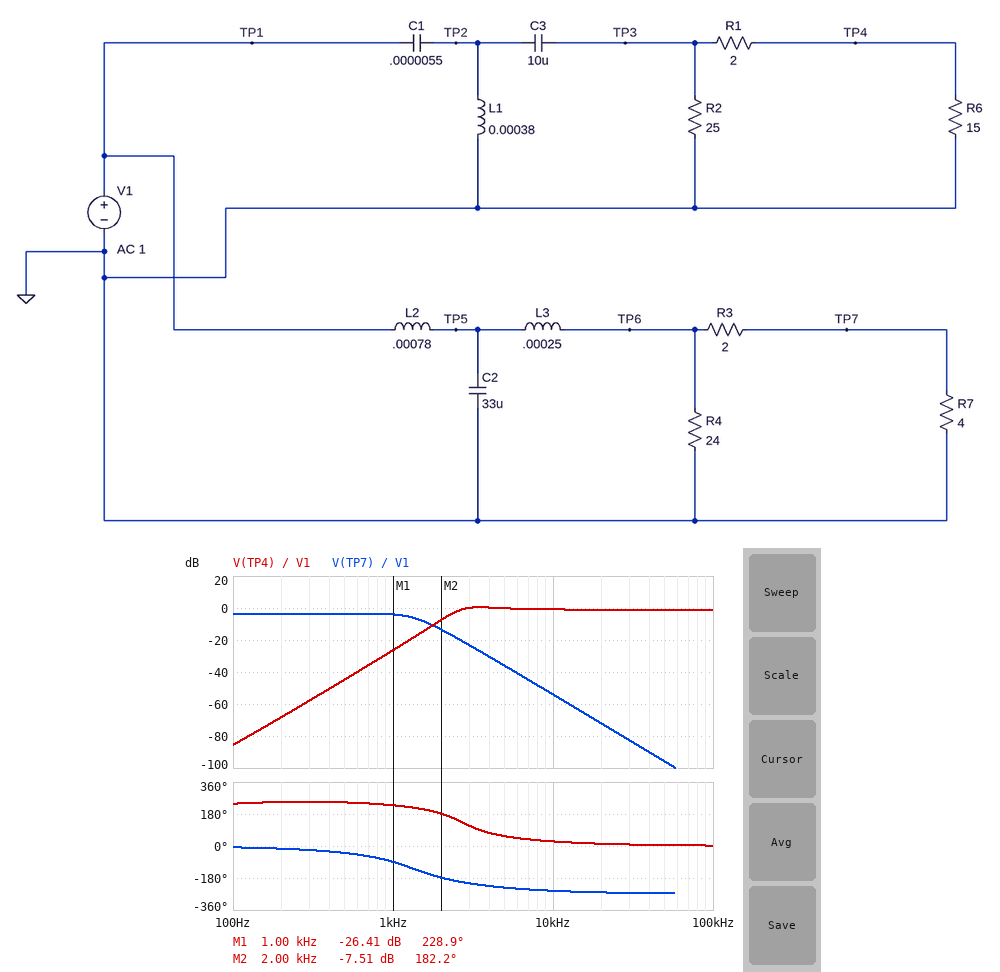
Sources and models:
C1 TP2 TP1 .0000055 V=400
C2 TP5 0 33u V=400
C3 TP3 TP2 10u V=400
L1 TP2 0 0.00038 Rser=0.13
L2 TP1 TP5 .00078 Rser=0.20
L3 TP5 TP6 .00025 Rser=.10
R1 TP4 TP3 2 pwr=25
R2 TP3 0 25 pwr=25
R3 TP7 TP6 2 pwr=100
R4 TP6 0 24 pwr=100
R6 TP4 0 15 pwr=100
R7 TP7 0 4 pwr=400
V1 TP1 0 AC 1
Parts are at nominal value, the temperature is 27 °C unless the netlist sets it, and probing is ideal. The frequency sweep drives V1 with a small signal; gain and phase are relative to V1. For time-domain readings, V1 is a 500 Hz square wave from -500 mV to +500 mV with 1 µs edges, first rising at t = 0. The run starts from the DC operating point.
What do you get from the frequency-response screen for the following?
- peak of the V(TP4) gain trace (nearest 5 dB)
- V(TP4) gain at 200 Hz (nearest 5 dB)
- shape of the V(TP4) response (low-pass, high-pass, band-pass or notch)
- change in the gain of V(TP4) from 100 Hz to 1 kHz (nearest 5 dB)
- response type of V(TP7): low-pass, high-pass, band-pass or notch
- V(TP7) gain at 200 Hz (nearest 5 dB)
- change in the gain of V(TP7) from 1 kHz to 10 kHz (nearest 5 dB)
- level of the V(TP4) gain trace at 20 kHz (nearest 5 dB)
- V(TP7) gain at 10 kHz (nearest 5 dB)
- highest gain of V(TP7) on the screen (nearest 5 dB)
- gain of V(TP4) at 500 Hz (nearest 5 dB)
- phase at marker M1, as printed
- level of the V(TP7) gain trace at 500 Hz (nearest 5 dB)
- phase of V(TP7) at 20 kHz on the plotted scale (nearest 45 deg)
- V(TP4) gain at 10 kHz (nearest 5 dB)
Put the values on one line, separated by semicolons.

0 dB; -70 dB; high-pass; 60 dB; low-pass; -5 dB; -50 dB; 0 dB; -55 dB; -5 dB; -45 dB; 228.9 deg; -5 dB; -270 deg; 0 dB
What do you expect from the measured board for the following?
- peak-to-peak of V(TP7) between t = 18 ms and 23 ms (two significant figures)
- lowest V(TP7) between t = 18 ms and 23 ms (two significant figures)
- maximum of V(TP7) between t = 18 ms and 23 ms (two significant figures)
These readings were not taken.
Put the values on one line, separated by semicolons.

770 mV; -380 mV; 380 mV
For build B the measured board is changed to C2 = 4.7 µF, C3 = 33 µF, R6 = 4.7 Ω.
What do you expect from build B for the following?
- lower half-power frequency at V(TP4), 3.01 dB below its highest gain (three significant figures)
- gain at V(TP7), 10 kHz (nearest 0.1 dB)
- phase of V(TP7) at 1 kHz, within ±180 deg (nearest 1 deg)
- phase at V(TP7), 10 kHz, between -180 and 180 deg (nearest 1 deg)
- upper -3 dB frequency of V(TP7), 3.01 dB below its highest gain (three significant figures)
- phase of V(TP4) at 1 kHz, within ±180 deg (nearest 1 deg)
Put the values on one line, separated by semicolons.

4.21 kHz; -34.8 dB; -55 deg; 112 deg; 887 Hz; -161 deg
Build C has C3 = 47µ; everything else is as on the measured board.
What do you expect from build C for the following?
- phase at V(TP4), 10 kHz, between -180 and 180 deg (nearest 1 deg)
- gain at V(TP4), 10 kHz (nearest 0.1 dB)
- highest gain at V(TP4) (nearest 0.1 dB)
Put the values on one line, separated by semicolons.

20 deg; -0.5 dB; 1.1 dB
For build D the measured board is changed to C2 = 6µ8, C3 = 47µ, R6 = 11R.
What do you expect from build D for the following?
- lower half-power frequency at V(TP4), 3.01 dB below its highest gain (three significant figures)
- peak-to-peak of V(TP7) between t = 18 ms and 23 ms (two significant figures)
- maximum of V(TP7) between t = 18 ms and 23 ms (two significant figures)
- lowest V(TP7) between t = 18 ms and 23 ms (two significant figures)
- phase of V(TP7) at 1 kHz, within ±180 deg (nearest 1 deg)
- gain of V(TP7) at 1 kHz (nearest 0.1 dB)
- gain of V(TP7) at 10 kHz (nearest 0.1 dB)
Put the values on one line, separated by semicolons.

2.84 kHz; 620 mV; 310 mV; -310 mV; -57 deg; -7.3 dB; -38.9 dB
